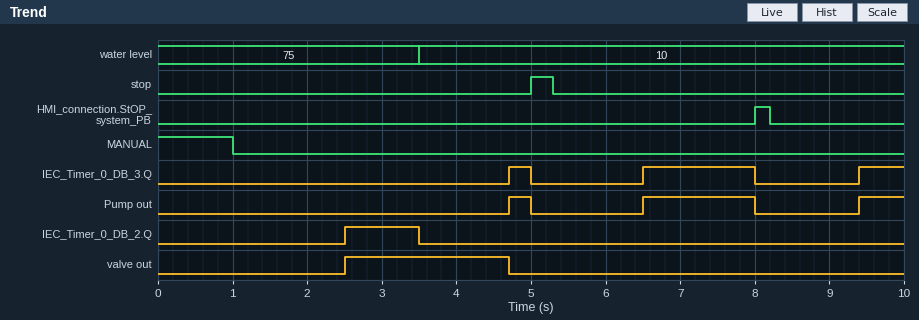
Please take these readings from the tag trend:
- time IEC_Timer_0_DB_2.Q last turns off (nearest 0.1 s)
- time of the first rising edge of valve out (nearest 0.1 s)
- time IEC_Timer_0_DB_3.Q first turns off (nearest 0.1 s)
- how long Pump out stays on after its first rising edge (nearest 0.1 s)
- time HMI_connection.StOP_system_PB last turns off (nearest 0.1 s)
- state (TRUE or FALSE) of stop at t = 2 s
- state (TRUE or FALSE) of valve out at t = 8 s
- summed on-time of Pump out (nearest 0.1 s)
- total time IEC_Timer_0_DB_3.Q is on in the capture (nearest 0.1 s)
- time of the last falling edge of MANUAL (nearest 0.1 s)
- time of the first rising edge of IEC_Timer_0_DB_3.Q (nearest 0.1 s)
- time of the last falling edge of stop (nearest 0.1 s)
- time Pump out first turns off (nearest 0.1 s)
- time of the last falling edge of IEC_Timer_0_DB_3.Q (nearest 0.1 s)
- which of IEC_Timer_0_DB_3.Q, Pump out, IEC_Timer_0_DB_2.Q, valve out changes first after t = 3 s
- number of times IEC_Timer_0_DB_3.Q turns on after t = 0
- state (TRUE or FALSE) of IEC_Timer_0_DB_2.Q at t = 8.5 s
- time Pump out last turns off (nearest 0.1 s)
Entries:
3.5 s
2.5 s
5.0 s
0.3 s
8.2 s
FALSE
FALSE
2.4 s
2.4 s
1.0 s
4.7 s
5.3 s
5.0 s
8.0 s
IEC_Timer_0_DB_2.Q
3
FALSE
8.0 s
